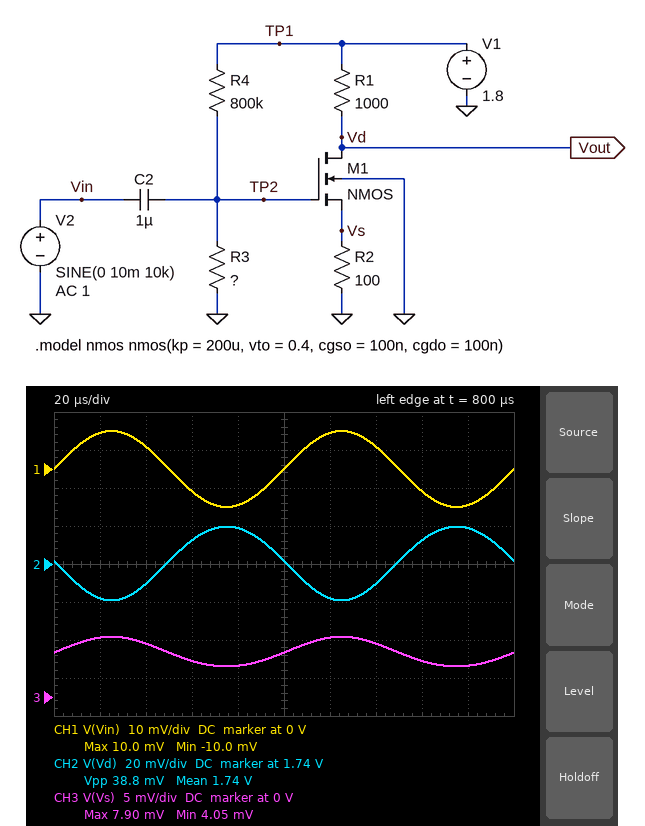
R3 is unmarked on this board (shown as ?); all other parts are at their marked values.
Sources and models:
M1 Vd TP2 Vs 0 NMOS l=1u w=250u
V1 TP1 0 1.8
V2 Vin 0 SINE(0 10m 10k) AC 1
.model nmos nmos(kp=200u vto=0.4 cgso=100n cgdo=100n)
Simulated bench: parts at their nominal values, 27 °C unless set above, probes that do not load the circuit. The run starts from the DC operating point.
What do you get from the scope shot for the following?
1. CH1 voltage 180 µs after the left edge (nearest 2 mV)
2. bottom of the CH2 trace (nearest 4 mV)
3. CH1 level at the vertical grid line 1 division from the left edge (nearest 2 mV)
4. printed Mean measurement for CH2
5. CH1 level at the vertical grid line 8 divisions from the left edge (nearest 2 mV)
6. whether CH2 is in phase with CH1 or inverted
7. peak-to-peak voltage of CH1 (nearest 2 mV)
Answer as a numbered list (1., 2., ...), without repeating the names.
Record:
1. -10 mV
2. 1.720 V
3. 10 mV
4. 1.74 V
5. -6 mV
6. inverted
7. 20 mV
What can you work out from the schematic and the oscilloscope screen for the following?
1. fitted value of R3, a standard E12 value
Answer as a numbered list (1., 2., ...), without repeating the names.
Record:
1. 270 kΩ
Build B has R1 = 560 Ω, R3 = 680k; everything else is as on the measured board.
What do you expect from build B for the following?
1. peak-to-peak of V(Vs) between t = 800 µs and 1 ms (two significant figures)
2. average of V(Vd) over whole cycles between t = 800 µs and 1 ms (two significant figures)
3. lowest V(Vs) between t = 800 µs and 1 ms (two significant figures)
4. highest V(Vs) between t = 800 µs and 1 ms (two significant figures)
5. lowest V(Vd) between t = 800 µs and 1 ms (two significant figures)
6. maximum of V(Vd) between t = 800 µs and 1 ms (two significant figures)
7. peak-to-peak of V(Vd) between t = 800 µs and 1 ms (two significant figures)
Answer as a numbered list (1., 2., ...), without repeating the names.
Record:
1. 11 mV
2. 860 mV
3. 160 mV
4. 170 mV
5. 830 mV
6. 890 mV
7. 63 mV
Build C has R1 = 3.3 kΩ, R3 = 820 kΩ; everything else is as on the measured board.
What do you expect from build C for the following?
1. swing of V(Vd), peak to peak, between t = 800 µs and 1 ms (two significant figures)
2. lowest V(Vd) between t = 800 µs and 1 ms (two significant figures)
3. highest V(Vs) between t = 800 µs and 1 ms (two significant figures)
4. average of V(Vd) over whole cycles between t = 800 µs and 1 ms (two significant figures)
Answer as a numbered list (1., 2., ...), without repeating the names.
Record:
1. 1.0 mV
2. 75 mV
3. 52 mV
4. 76 mV
